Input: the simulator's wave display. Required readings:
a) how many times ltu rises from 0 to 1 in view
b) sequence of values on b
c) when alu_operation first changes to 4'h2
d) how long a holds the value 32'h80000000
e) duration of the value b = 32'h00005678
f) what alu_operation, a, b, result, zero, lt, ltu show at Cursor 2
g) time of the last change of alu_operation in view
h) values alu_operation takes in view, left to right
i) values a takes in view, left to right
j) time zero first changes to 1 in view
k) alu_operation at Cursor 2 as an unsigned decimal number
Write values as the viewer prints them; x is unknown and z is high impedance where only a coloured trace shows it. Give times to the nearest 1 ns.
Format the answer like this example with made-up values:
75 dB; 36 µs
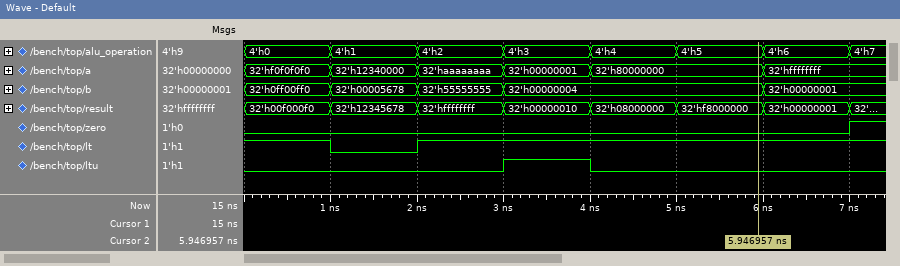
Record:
1; 32'h0ff00ff0, 32'h00005678, 32'h55555555, 32'h00000004, 32'h00000001; 2 ns; 2 ns; 1 ns; alu_operation=4'h5, a=32'h80000000, b=32'h00000004, result=32'hf8000000, zero=0, lt=1, ltu=0; 7 ns; 4'h0, 4'h1, 4'h2, 4'h3, 4'h4, 4'h5, 4'h6, 4'h7; 32'hf0f0f0f0, 32'h12340000, 32'haaaaaaaa, 32'h00000001, 32'h80000000, 32'hffffffff; 7 ns; 5
